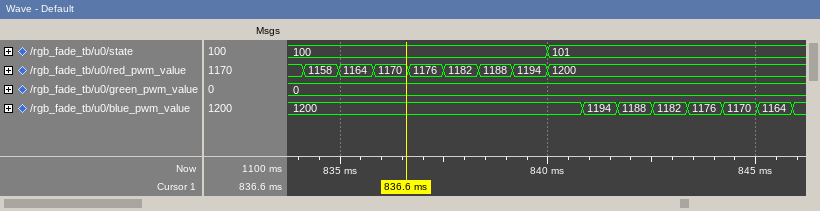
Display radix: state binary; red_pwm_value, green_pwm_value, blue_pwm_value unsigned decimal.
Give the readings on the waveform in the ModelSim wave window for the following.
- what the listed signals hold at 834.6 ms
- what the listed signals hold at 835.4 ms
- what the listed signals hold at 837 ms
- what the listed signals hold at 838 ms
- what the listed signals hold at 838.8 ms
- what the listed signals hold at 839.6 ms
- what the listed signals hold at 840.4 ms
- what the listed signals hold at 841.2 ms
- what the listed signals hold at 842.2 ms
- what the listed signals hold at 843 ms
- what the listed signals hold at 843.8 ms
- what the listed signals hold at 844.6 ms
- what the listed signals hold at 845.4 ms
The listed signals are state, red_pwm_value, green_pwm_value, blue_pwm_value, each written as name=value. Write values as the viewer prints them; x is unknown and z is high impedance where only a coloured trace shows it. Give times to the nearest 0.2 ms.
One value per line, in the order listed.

state=100, red_pwm_value=1158, green_pwm_value=0, blue_pwm_value=1200
state=100, red_pwm_value=1164, green_pwm_value=0, blue_pwm_value=1200
state=100, red_pwm_value=1176, green_pwm_value=0, blue_pwm_value=1200
state=100, red_pwm_value=1182, green_pwm_value=0, blue_pwm_value=1200
state=100, red_pwm_value=1188, green_pwm_value=0, blue_pwm_value=1200
state=100, red_pwm_value=1194, green_pwm_value=0, blue_pwm_value=1200
state=101, red_pwm_value=1200, green_pwm_value=0, blue_pwm_value=1200
state=101, red_pwm_value=1200, green_pwm_value=0, blue_pwm_value=1194
state=101, red_pwm_value=1200, green_pwm_value=0, blue_pwm_value=1188
state=101, red_pwm_value=1200, green_pwm_value=0, blue_pwm_value=1182
state=101, red_pwm_value=1200, green_pwm_value=0, blue_pwm_value=1176
state=101, red_pwm_value=1200, green_pwm_value=0, blue_pwm_value=1170
state=101, red_pwm_value=1200, green_pwm_value=0, blue_pwm_value=1164
